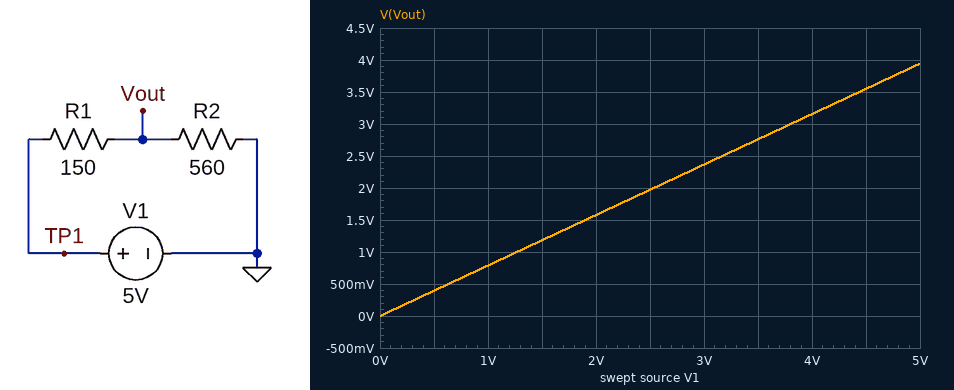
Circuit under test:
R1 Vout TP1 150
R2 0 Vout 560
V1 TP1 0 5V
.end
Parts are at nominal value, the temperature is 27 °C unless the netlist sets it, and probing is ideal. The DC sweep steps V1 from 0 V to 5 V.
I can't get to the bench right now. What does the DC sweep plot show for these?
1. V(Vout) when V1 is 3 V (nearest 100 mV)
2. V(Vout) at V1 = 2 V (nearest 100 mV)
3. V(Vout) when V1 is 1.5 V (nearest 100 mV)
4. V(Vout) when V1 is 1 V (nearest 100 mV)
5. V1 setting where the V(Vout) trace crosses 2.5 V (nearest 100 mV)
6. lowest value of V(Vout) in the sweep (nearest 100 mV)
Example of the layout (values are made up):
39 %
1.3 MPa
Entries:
2.4 V
1.6 V
1.2 V
800 mV
3.2 V
0 V
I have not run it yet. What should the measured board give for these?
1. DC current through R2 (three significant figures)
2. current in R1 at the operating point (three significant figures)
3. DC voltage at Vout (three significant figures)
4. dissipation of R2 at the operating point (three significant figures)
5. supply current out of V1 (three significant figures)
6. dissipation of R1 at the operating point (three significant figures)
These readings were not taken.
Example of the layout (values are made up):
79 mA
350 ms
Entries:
7.04 mA
7.04 mA
3.94 V
27.8 mW
7.04 mA
7.44 mW
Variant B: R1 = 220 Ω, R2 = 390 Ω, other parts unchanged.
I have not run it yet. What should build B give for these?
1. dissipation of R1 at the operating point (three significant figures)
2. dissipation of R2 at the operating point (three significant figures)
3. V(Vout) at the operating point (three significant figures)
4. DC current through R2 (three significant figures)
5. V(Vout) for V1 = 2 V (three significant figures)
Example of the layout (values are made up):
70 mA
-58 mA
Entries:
14.8 mW
26.2 mW
3.20 V
8.20 mA
1.28 V
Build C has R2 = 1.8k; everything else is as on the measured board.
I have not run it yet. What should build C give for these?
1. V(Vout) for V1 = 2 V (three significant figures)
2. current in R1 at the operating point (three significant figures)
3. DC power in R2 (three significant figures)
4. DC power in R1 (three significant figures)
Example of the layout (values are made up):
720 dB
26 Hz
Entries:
1.85 V
2.56 mA
11.8 mW
986 µW
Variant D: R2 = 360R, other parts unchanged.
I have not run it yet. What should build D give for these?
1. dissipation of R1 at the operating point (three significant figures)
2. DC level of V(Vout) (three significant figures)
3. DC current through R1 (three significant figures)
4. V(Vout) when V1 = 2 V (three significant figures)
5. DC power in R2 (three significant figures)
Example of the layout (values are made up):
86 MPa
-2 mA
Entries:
14.4 mW
3.53 V
9.80 mA
1.41 V
34.6 mW
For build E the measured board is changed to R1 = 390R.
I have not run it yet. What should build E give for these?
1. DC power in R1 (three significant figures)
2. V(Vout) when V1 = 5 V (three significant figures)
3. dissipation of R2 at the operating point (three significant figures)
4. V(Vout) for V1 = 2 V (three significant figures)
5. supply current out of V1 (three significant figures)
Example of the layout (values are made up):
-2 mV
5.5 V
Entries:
10.8 mW
2.95 V
15.5 mW
1.18 V
5.26 mA
